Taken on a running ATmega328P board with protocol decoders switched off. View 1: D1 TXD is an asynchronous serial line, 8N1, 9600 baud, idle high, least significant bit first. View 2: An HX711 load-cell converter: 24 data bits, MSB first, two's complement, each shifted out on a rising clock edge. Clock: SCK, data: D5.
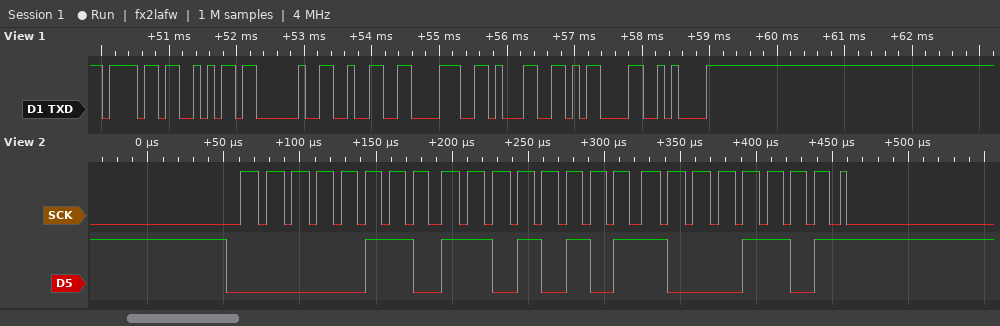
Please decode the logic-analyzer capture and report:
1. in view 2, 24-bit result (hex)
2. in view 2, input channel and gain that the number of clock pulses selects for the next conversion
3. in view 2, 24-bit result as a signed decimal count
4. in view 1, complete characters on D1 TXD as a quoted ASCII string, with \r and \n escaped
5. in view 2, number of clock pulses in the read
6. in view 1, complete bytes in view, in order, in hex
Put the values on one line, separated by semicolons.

0x06D58D; channel A, gain 128; 447885; "oj 281\r\n"; 25; 6F 6A 20 32 38 31 0D 0A
